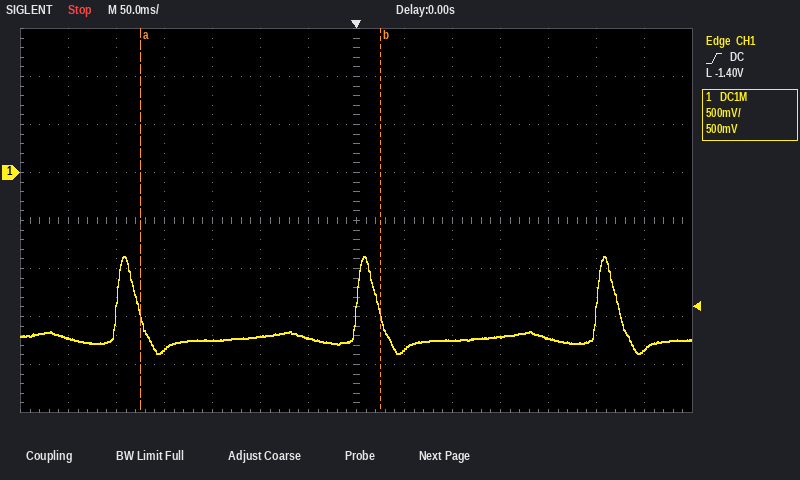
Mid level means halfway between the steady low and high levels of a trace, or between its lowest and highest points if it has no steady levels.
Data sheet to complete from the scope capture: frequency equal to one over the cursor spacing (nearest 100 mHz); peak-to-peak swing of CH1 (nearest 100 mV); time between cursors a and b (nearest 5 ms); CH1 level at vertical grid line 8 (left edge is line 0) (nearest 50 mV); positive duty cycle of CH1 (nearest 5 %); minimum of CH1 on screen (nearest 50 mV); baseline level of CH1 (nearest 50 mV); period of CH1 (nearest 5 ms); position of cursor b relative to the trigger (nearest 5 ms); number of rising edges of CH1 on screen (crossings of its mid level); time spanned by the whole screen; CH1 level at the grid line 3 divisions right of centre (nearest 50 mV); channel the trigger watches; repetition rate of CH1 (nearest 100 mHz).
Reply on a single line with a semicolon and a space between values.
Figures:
4.0 Hz; 1.00 V; 250 ms; -1.85 V; 10 %; -1.90 V; -1.75 V; 250 ms; +25 ms; 3; 700 ms; -1.70 V; CH1; 4.0 Hz
